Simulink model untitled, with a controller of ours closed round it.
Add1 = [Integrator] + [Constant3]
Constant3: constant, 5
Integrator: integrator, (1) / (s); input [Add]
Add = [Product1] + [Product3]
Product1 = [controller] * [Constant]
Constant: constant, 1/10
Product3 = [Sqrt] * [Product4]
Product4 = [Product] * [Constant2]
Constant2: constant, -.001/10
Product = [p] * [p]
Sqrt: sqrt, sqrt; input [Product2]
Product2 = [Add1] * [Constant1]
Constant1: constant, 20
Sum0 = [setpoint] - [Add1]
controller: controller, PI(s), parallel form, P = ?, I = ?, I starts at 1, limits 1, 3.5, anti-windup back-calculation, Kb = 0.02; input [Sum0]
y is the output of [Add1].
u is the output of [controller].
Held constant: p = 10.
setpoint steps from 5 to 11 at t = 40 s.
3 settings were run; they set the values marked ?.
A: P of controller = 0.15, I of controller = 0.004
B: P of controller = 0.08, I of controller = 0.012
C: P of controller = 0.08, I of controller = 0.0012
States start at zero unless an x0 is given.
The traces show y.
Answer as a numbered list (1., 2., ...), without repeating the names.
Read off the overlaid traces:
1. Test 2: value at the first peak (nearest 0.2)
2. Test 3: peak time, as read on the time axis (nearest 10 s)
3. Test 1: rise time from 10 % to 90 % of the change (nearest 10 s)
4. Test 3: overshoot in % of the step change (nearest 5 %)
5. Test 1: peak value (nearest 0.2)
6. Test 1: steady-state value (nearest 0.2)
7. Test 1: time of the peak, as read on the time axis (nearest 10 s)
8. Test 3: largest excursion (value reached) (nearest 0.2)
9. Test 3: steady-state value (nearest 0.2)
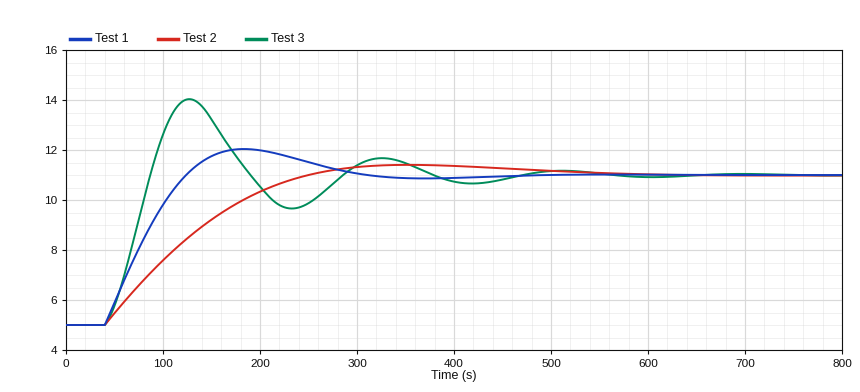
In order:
1. 11.4
2. 130 s
3. 60 s
4. 50 %
5. 12.0
6. 11.0
7. 180 s
8. 14.0
9. 11.0
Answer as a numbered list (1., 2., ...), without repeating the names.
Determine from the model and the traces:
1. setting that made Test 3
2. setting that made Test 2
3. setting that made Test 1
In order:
1. B
2. C
3. A
